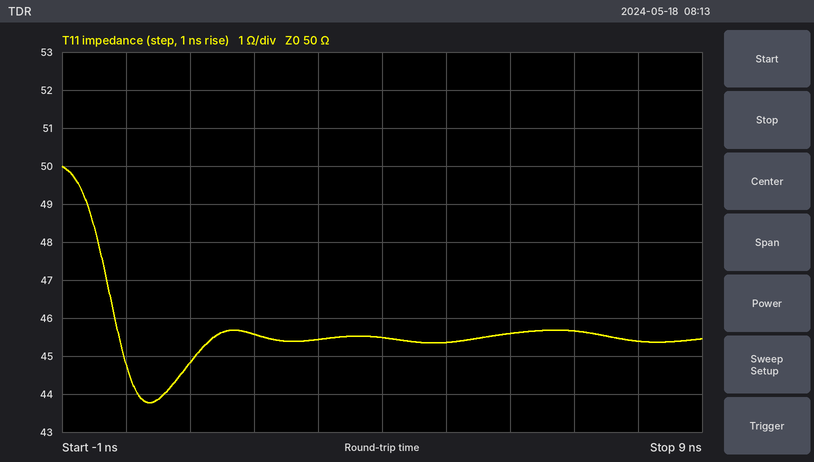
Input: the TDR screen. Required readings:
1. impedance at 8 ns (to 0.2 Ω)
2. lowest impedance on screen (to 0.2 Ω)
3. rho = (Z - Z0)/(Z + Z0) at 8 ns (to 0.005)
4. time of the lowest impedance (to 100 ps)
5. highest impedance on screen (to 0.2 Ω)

45.4 Ω
43.8 Ω
-0.050
400 ps
50.0 Ω
